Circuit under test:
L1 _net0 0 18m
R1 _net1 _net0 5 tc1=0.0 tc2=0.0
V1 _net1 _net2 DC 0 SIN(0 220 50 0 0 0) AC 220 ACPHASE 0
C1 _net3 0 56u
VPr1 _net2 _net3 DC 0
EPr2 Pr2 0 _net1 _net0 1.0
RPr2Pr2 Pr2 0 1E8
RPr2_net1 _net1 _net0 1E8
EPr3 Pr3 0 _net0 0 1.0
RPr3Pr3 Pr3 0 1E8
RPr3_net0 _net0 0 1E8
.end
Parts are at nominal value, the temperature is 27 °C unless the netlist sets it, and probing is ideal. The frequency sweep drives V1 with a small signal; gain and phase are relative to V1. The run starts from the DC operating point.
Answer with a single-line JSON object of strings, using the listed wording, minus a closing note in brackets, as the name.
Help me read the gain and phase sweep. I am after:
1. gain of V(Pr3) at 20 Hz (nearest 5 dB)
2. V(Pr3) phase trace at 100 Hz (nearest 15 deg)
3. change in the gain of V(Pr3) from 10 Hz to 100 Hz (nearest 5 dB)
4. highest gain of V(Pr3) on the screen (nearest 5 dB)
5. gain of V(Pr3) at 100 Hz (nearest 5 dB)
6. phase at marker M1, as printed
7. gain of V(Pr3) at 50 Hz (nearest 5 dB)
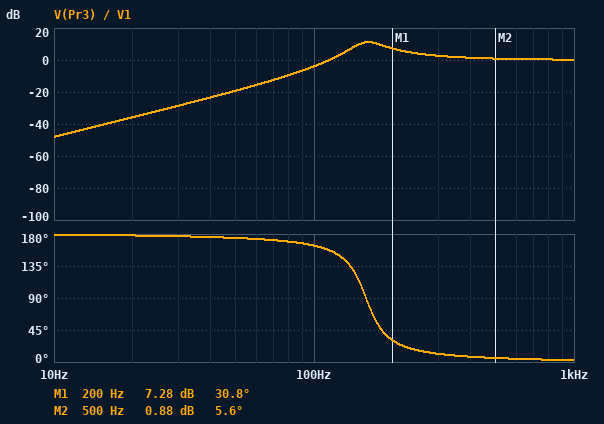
{"gain of V(Pr3) at 20 Hz": "-35 dB", "V(Pr3) phase trace at 100 Hz": "165 deg", "change in the gain of V(Pr3) from 10 Hz to 100 Hz": "45 dB", "highest gain of V(Pr3) on the screen": "10 dB", "gain of V(Pr3) at 100 Hz": "-5 dB", "phase at marker M1, as printed": "30.8 deg", "gain of V(Pr3) at 50 Hz": "-20 dB"}
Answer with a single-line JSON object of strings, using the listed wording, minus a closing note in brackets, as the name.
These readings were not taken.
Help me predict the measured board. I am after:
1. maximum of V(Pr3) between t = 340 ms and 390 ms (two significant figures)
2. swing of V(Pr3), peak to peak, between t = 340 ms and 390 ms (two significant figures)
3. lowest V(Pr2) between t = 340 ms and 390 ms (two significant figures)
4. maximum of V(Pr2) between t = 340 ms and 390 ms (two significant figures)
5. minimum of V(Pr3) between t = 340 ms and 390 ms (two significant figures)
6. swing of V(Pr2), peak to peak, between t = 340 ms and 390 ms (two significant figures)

{"maximum of V(Pr3) between t = 340 ms and 390 ms": "24 V", "swing of V(Pr3), peak to peak, between t = 340 ms and 390 ms": "48 V", "lowest V(Pr2) between t = 340 ms and 390 ms": "-21 V", "maximum of V(Pr2) between t = 340 ms and 390 ms": "21 V", "minimum of V(Pr3) between t = 340 ms and 390 ms": "-24 V", "swing of V(Pr2), peak to peak, between t = 340 ms and 390 ms": "43 V"}
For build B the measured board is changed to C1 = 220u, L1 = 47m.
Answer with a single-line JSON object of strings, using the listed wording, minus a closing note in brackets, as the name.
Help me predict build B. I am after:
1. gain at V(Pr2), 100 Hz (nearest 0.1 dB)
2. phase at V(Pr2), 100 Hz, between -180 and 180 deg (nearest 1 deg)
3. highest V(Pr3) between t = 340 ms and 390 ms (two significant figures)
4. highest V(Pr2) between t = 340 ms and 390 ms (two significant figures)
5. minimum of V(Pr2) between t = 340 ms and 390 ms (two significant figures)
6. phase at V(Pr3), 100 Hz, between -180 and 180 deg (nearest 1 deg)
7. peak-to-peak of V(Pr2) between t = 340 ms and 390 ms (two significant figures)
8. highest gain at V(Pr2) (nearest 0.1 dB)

{"gain at V(Pr2), 100 Hz": "-13.2 dB", "phase at V(Pr2), 100 Hz, between -180 and 180 deg": "-77 deg", "highest V(Pr3) between t = 340 ms and 390 ms": "650 V", "highest V(Pr2) between t = 340 ms and 390 ms": "220 V", "minimum of V(Pr2) between t = 340 ms and 390 ms": "-220 V", "phase at V(Pr3), 100 Hz, between -180 and 180 deg": "13 deg", "peak-to-peak of V(Pr2) between t = 340 ms and 390 ms": "440 V", "highest gain at V(Pr2)": "0 dB"}
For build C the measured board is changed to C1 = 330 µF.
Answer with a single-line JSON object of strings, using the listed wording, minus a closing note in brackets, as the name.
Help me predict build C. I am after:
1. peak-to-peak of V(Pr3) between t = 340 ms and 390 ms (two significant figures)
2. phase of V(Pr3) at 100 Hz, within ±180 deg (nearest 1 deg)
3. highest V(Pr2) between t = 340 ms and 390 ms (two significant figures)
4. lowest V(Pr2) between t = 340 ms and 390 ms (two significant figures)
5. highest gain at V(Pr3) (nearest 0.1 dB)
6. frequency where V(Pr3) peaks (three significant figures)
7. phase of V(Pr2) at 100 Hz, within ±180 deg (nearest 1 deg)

{"peak-to-peak of V(Pr3) between t = 340 ms and 390 ms": "390 V", "phase of V(Pr3) at 100 Hz, within ±180 deg": "38 deg", "highest V(Pr2) between t = 340 ms and 390 ms": "170 V", "lowest V(Pr2) between t = 340 ms and 390 ms": "-170 V", "highest gain at V(Pr3)": "3.9 dB", "frequency where V(Pr3) peaks": "74.4 Hz", "phase of V(Pr2) at 100 Hz, within ±180 deg": "-52 deg"}
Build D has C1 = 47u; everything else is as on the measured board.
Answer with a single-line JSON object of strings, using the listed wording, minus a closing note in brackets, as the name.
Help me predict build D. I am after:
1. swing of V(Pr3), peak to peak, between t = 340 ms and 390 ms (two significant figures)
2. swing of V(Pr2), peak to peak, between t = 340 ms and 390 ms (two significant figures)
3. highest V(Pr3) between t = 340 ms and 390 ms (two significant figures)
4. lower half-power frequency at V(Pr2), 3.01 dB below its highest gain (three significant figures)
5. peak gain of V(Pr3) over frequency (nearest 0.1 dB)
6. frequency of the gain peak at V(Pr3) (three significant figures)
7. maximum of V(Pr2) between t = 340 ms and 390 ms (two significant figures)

{"swing of V(Pr3), peak to peak, between t = 340 ms and 390 ms": "40 V", "swing of V(Pr2), peak to peak, between t = 340 ms and 390 ms": "35 V", "highest V(Pr3) between t = 340 ms and 390 ms": "20 V", "lower half-power frequency at V(Pr2), 3.01 dB below its highest gain": "152 Hz", "peak gain of V(Pr3) over frequency": "11.9 dB", "frequency of the gain peak at V(Pr3)": "176 Hz", "maximum of V(Pr2) between t = 340 ms and 390 ms": "18 V"}
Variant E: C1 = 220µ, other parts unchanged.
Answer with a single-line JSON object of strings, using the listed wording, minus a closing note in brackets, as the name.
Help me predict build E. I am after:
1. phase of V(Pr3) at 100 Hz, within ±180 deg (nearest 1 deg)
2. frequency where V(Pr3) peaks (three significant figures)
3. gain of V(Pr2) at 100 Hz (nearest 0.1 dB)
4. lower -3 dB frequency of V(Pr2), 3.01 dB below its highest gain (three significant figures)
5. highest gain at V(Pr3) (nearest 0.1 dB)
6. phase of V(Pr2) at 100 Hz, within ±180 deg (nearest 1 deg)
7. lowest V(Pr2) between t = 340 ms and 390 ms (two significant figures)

{"phase of V(Pr3) at 100 Hz, within ±180 deg": "51 deg", "frequency where V(Pr3) peaks": "86.9 Hz", "gain of V(Pr2) at 100 Hz": "-2.2 dB", "lower -3 dB frequency of V(Pr2), 3.01 dB below its highest gain": "60.9 Hz", "highest gain at V(Pr3)": "5.5 dB", "phase of V(Pr2) at 100 Hz, within ±180 deg": "-39 deg", "lowest V(Pr2) between t = 340 ms and 390 ms": "-110 V"}
